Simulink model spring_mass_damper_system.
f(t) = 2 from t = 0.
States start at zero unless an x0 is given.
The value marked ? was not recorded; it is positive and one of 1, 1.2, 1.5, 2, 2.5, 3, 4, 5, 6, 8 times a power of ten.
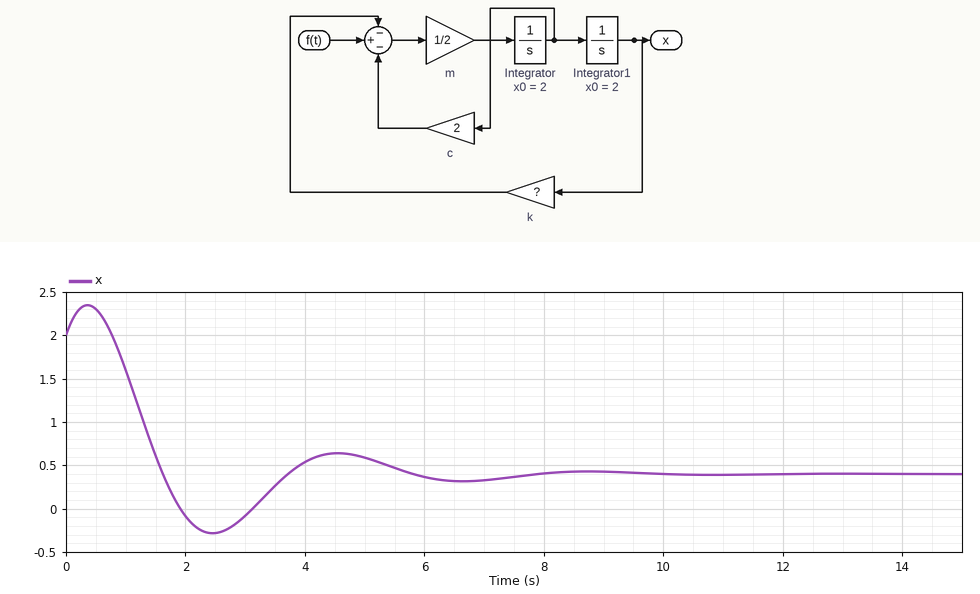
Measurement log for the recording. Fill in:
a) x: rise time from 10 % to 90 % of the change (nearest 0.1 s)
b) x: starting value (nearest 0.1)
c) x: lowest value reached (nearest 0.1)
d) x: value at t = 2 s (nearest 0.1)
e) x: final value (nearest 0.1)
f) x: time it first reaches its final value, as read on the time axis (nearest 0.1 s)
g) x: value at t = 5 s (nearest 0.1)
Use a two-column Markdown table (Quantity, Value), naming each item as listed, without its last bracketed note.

| Quantity | Value |
|---|---|
| x: rise time from 10 % to 90 % of the change | 0.7 s |
| x: starting value | 2.0 |
| x: lowest value reached | -0.3 |
| x: value at t = 2 s | -0.1 |
| x: final value | 0.4 |
| x: time it first reaches its final value, as read on the time axis | 1.6 s |
| x: value at t = 5 s | 0.6 |
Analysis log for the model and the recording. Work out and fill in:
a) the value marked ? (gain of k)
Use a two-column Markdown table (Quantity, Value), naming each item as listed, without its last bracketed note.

| Quantity | Value |
|---|---|
| the value marked ? | 5 |
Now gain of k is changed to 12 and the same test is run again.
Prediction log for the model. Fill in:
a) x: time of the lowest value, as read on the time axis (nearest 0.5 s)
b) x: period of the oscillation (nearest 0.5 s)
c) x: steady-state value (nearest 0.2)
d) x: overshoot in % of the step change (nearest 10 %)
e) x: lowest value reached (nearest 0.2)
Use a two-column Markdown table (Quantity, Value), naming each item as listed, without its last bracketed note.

| Quantity | Value |
|---|---|
| x: time of the lowest value, as read on the time axis | 1.5 s |
| x: period of the oscillation | 2.5 s |
| x: steady-state value | 0.2 |
| x: overshoot in % of the step change | 60 % |
| x: lowest value reached | -0.8 |
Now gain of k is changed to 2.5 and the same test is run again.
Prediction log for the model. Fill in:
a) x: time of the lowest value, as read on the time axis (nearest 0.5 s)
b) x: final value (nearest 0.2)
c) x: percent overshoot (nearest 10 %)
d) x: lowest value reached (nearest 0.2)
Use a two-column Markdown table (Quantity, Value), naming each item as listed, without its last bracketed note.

| Quantity | Value |
|---|---|
| x: time of the lowest value, as read on the time axis | 4.0 s |
| x: final value | 0.8 |
| x: percent overshoot | 30 % |
| x: lowest value reached | 0.4 |
